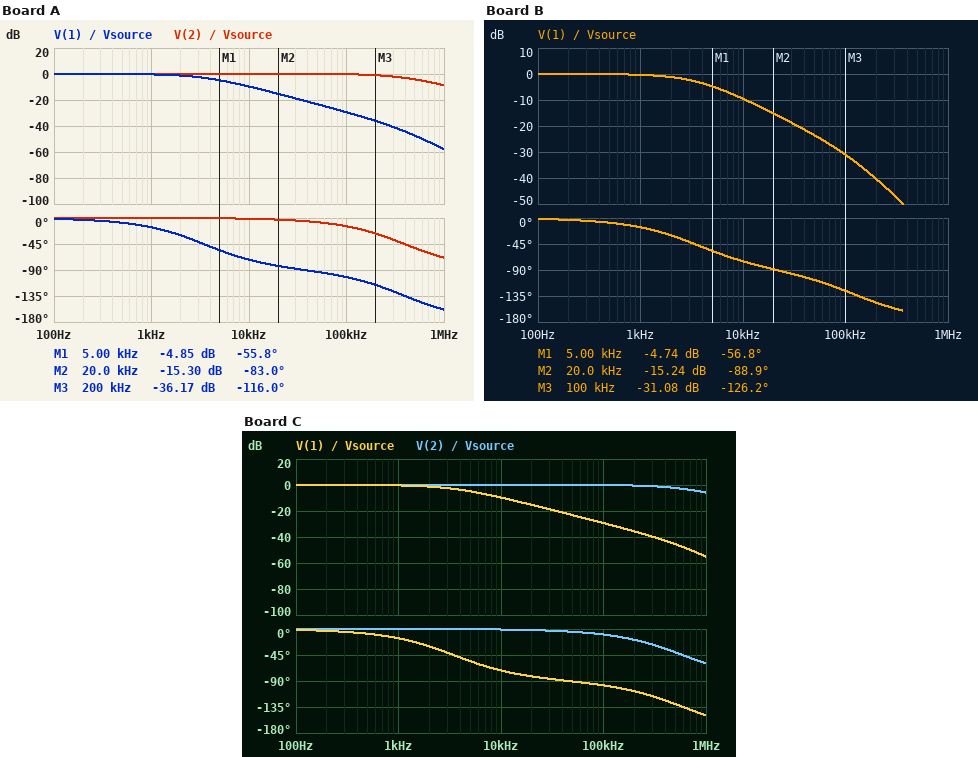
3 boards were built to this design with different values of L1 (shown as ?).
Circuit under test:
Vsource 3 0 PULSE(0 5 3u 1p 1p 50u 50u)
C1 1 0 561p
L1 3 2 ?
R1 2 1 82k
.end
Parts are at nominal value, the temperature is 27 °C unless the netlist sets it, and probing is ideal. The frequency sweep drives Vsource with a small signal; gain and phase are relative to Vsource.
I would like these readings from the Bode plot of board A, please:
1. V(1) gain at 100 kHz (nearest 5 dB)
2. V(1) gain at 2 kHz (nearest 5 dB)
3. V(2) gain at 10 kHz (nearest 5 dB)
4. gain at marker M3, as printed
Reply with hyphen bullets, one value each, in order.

- -30 dB
- 0 dB
- 0 dB
- -36.17 dB
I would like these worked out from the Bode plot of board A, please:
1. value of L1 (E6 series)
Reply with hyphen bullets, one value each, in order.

- 33 mH
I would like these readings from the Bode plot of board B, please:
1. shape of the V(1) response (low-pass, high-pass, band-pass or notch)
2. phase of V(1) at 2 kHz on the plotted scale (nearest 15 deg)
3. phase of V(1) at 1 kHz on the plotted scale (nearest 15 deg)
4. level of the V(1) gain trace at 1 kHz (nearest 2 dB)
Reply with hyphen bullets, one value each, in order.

- low-pass
- -30 deg
- -15 deg
- 0 dB
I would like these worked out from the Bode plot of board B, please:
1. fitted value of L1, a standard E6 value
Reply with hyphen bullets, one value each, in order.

- 100 mH
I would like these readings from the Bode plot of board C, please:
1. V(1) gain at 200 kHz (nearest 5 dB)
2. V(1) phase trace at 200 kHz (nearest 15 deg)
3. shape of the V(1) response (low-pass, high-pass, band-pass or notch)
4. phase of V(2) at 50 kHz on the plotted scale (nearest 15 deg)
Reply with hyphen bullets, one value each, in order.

- -35 dB
- -105 deg
- low-pass
- 0 deg
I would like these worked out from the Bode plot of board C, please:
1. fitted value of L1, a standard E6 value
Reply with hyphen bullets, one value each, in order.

- 22 mH
